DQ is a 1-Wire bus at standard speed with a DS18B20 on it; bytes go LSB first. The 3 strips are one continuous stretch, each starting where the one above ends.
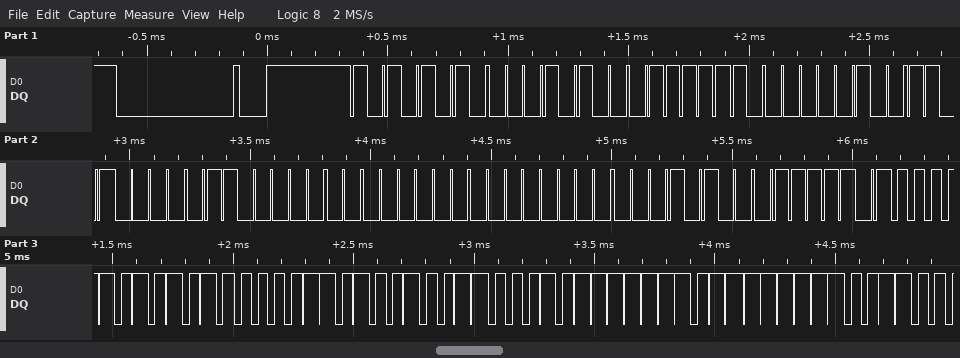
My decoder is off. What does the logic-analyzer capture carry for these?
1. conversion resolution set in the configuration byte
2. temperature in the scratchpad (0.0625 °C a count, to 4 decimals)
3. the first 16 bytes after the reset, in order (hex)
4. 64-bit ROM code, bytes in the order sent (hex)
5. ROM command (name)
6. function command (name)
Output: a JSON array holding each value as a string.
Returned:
["12 bits", "85.0000 °C", "55 28 7E 20 0B 06 00 00 28 BE 50 05 4B 46 7F FF", "28 7E 20 0B 06 00 00 28", "Match ROM", "Read Scratchpad"]
